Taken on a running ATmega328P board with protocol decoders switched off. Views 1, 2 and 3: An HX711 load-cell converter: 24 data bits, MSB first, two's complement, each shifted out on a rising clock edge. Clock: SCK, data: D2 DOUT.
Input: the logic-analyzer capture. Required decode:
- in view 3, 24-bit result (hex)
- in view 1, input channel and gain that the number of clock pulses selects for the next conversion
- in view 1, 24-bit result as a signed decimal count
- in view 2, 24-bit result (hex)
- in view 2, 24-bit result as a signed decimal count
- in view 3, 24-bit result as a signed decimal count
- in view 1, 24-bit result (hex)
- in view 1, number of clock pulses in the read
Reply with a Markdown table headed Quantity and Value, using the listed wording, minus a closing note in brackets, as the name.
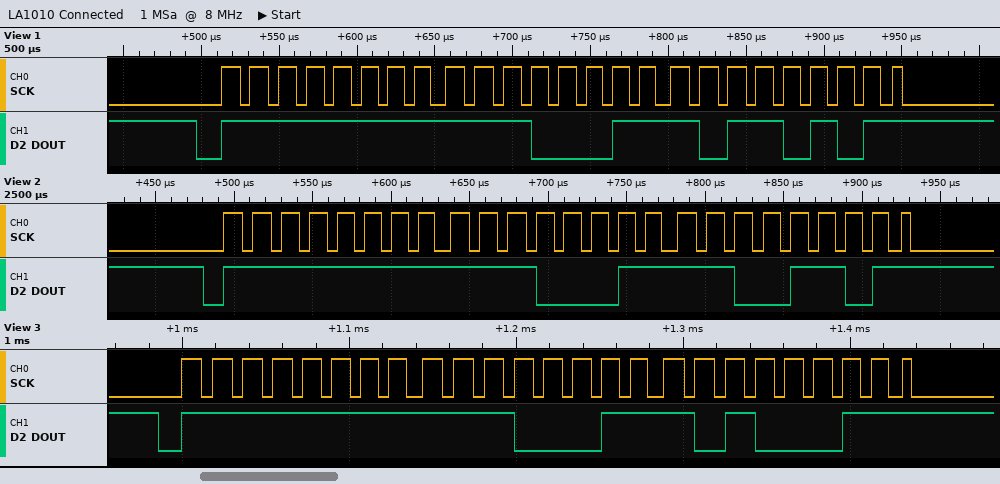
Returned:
| Quantity | Value |
|---|---|
| in view 3, 24-bit result | 0xFFE3A3 |
| in view 1, input channel and gain that the number of clock pulses selects for the next conversion | channel A, gain 128 |
| in view 1, 24-bit result as a signed decimal count | -7243 |
| in view 2, 24-bit result | 0xFFE3CD |
| in view 2, 24-bit result as a signed decimal count | -7219 |
| in view 3, 24-bit result as a signed decimal count | -7261 |
| in view 1, 24-bit result | 0xFFE3B5 |
| in view 1, number of clock pulses in the read | 25 |
